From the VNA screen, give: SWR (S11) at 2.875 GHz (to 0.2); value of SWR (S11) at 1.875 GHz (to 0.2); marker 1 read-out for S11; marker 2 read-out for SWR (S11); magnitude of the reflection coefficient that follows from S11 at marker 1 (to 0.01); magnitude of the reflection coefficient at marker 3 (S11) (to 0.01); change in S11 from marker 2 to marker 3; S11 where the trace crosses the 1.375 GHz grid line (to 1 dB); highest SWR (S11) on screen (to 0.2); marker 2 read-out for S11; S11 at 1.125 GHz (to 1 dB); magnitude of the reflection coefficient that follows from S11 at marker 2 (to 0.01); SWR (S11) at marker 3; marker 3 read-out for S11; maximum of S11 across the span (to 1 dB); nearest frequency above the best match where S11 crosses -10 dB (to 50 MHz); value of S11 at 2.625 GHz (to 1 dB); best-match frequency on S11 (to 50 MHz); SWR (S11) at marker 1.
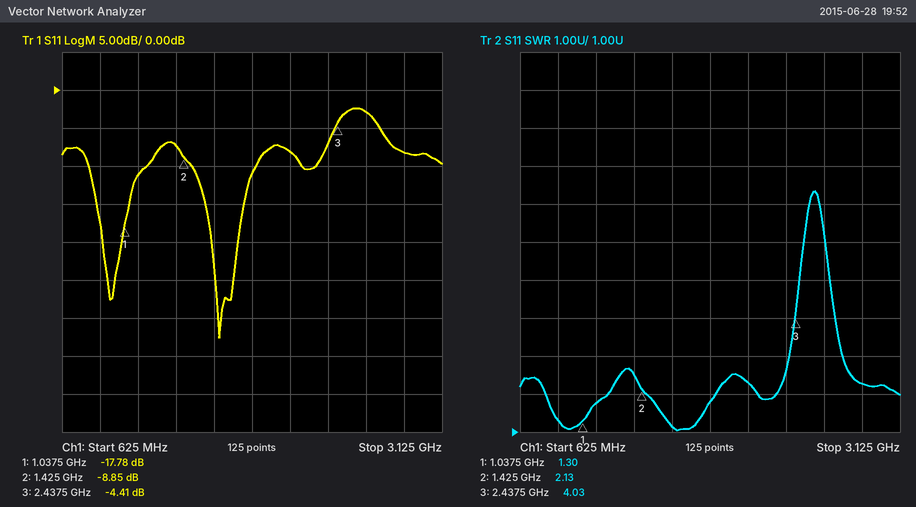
2.2
1.8
-17.78 dB
2.13
0.13
0.60
4.44 dB
-7 dB
7.4
-8.85 dB
-11 dB
0.36
4.03
-4.41 dB
-2 dB
1.90 GHz
-3 dB
1.65 GHz
1.30
